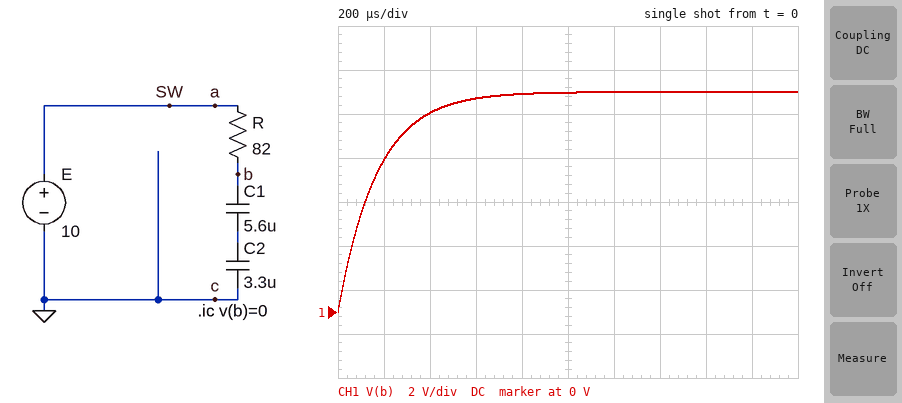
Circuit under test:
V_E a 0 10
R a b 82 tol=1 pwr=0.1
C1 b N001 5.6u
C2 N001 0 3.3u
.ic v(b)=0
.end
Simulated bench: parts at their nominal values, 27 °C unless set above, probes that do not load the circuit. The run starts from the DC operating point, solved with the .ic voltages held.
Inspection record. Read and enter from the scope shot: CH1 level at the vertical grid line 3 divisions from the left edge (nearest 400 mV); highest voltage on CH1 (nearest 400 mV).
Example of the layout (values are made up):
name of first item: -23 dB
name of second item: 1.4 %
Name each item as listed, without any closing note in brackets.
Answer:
CH1 level at the vertical grid line 3 divisions from the left edge: 9.6 V
highest voltage on CH1: 10.0 V
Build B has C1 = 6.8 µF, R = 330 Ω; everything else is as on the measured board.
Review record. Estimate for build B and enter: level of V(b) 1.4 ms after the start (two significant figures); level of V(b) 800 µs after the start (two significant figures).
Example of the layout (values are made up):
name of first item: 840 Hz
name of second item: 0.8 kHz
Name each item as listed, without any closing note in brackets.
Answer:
level of V(b) 1.4 ms after the start: 8.5 V
level of V(b) 800 µs after the start: 6.6 V
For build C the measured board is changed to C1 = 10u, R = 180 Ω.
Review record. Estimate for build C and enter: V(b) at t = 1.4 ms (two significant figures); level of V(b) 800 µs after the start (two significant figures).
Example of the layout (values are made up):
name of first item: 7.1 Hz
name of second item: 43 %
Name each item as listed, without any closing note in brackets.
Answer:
V(b) at t = 1.4 ms: 9.6 V
level of V(b) 800 µs after the start: 8.3 V
